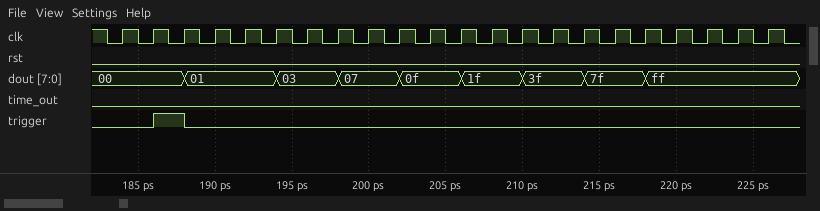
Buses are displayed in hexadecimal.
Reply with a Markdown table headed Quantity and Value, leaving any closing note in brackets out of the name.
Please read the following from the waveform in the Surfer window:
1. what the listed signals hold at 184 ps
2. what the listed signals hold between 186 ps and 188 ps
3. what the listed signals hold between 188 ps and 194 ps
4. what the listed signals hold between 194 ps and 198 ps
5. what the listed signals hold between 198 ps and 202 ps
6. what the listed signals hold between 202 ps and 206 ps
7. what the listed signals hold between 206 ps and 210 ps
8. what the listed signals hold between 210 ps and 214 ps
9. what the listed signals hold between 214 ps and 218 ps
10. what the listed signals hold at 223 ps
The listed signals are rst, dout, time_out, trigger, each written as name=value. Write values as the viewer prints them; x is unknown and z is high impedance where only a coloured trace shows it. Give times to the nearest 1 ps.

| Quantity | Value |
|---|---|
| what the listed signals hold at 184 ps | rst=0, dout=00, time_out=0, trigger=0 |
| what the listed signals hold between 186 ps and 188 ps | rst=0, dout=00, time_out=0, trigger=1 |
| what the listed signals hold between 188 ps and 194 ps | rst=0, dout=01, time_out=0, trigger=0 |
| what the listed signals hold between 194 ps and 198 ps | rst=0, dout=03, time_out=0, trigger=0 |
| what the listed signals hold between 198 ps and 202 ps | rst=0, dout=07, time_out=0, trigger=0 |
| what the listed signals hold between 202 ps and 206 ps | rst=0, dout=0f, time_out=0, trigger=0 |
| what the listed signals hold between 206 ps and 210 ps | rst=0, dout=1f, time_out=0, trigger=0 |
| what the listed signals hold between 210 ps and 214 ps | rst=0, dout=3f, time_out=0, trigger=0 |
| what the listed signals hold between 214 ps and 218 ps | rst=0, dout=7f, time_out=0, trigger=0 |
| what the listed signals hold at 223 ps | rst=0, dout=ff, time_out=0, trigger=0 |
